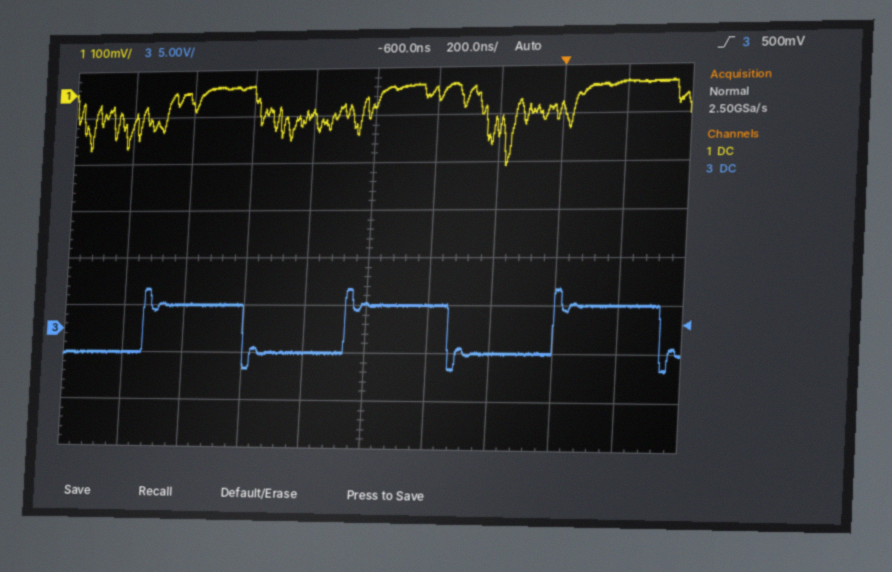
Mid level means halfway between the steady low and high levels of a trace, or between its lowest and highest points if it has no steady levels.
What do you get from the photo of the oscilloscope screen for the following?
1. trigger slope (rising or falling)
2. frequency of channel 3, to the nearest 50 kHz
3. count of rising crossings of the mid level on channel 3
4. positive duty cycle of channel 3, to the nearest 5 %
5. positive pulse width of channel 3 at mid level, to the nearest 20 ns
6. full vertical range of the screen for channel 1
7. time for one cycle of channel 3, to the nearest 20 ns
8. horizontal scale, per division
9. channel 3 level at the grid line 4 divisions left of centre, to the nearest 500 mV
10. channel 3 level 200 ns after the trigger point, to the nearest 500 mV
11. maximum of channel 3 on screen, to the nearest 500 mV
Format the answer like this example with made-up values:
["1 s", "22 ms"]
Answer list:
["rising", "1.50 MHz", "3", "50 %", "340 ns", "800 mV", "660 ns", "200 ns", "-2.5 V", "2.5 V", "4.5 V"]
